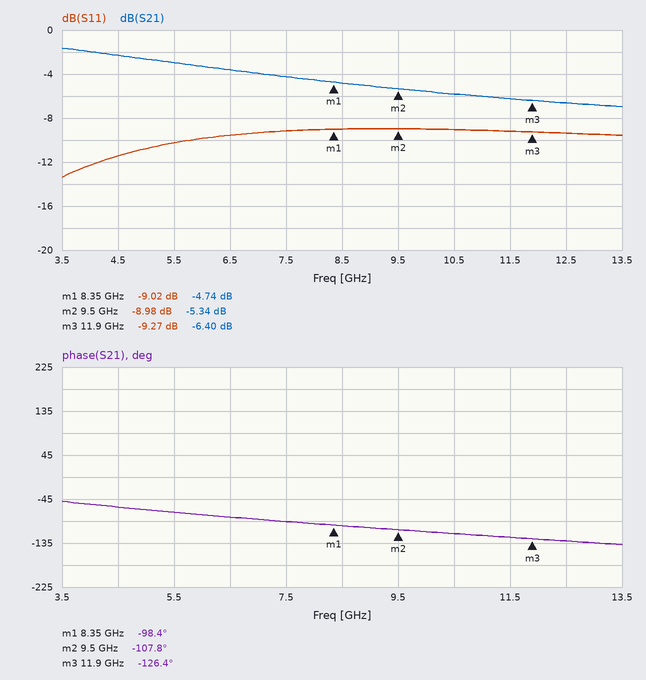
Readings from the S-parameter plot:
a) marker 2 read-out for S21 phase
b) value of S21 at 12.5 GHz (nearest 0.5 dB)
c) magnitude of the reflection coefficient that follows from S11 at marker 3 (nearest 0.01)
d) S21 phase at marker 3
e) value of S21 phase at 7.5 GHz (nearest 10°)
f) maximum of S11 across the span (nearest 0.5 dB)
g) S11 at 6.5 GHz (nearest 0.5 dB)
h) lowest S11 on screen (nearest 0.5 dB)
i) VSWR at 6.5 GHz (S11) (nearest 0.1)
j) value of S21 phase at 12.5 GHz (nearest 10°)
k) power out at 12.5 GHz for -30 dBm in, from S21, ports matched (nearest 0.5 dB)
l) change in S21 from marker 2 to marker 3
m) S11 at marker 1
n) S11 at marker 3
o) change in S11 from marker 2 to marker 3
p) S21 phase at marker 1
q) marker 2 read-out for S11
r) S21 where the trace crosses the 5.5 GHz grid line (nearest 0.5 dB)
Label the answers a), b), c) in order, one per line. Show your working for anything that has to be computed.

a) -107.8°
b) -6.5 dB
c) 10^(-9.27/20) ≈ 0.34
d) -126.4°
e) -90°
f) -9.0 dB
g) -9.5 dB
h) -13.5 dB
i) |Γ| = 10^(-9.5/20) = 0.3350; VSWR = (1 + 0.3350)/(1 − 0.3350) ≈ 2.0
j) -130°
k) -30 dBm + (-6.5 dB) = -36.5 dBm
l) -6.4 − (-5.34) = -1.06 dB
m) -9.02 dB
n) -9.27 dB
o) -9.27 − (-8.98) = -0.29 dB
p) -98.4°
q) -8.98 dB
r) -3.0 dB
